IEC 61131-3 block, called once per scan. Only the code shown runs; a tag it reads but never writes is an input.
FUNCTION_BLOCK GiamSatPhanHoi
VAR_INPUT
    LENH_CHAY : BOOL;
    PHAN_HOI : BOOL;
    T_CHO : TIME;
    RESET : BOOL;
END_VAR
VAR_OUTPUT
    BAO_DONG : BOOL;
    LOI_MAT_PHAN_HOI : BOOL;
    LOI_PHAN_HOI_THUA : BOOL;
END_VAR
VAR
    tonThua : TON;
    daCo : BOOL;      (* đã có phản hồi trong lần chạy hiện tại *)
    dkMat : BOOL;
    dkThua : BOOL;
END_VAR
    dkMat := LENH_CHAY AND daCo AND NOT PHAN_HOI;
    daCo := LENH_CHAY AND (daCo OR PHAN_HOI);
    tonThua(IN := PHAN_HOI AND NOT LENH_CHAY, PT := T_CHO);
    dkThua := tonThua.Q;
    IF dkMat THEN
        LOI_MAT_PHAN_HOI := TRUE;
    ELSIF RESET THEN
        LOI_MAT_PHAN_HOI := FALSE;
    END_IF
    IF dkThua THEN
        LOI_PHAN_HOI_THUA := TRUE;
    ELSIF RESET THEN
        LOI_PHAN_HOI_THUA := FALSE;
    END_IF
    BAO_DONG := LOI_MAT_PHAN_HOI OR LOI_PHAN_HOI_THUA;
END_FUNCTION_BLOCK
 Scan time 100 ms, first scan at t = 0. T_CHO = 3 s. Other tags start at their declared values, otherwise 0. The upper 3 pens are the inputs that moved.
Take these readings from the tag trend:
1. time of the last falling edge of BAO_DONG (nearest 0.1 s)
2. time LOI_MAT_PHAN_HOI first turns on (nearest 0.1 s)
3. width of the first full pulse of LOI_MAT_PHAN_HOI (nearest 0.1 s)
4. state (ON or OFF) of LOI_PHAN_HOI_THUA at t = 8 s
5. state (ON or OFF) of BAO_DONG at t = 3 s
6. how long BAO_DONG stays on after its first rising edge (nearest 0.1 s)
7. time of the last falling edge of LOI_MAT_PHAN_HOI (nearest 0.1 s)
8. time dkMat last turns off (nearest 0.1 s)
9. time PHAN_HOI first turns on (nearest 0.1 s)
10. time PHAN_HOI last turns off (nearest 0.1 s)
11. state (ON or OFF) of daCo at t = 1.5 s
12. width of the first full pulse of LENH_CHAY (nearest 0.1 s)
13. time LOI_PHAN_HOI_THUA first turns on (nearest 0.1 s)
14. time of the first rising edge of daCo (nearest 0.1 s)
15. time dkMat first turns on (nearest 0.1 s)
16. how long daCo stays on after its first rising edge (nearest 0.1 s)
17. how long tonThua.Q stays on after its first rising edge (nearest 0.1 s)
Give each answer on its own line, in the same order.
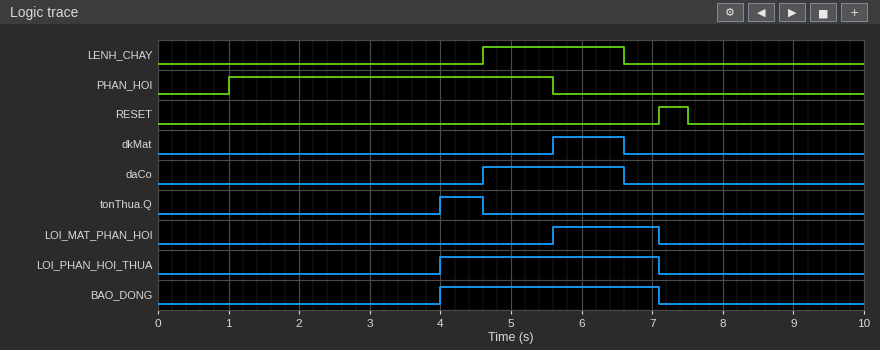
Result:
7.1 s
5.6 s
1.5 s
OFF
OFF
3.1 s
7.1 s
6.6 s
1.0 s
5.6 s
OFF
2.0 s
4.0 s
4.6 s
5.6 s
2.0 s
0.6 s
